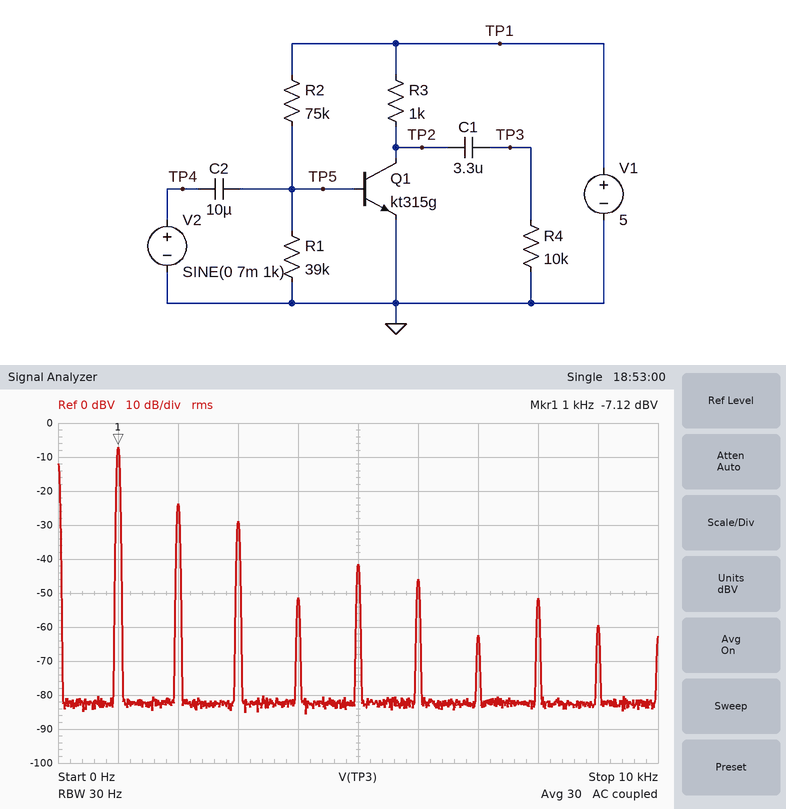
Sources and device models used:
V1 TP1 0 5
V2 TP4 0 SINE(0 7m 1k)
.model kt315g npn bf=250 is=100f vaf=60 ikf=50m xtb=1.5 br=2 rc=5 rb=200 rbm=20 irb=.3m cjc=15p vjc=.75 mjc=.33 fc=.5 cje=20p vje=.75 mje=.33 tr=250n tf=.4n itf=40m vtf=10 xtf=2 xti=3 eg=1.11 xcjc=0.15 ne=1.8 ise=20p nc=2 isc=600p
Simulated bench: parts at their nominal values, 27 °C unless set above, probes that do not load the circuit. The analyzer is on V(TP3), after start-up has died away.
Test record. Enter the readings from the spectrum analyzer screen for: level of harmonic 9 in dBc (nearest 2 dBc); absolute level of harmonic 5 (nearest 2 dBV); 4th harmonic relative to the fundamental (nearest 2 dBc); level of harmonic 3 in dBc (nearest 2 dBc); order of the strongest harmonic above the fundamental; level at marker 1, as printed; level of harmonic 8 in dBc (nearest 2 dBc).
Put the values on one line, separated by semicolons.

-52 dBc; -42 dBV; -44 dBc; -22 dBc; 2; -7.12 dBV; -44 dBc
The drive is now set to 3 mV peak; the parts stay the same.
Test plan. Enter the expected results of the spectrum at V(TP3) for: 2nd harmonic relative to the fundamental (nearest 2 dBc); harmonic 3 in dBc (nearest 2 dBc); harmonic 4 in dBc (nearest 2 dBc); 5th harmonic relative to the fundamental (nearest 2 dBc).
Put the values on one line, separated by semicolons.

-14 dBc; -26 dBc; -36 dBc; -38 dBc
